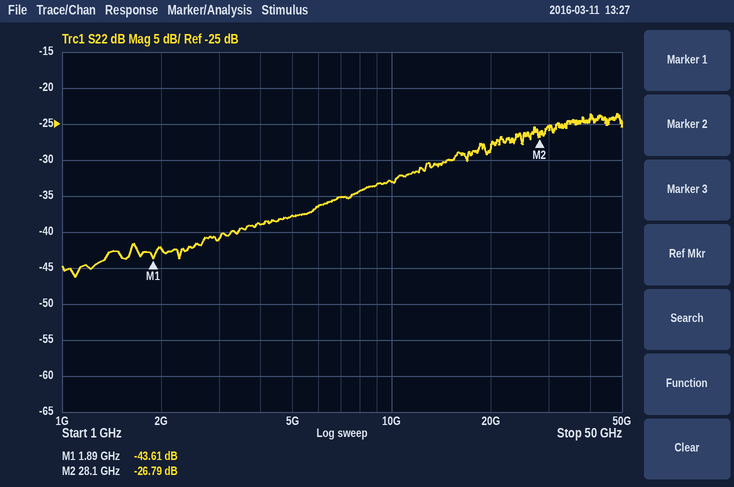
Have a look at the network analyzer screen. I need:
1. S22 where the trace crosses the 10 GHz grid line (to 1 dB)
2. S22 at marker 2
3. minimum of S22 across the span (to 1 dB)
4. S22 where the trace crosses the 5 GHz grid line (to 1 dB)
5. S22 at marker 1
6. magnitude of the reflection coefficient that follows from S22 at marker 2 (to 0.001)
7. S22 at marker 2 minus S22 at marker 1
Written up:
-33 dB
-26.79 dB
-46 dB
-38 dB
-43.61 dB
0.046
16.82 dB
